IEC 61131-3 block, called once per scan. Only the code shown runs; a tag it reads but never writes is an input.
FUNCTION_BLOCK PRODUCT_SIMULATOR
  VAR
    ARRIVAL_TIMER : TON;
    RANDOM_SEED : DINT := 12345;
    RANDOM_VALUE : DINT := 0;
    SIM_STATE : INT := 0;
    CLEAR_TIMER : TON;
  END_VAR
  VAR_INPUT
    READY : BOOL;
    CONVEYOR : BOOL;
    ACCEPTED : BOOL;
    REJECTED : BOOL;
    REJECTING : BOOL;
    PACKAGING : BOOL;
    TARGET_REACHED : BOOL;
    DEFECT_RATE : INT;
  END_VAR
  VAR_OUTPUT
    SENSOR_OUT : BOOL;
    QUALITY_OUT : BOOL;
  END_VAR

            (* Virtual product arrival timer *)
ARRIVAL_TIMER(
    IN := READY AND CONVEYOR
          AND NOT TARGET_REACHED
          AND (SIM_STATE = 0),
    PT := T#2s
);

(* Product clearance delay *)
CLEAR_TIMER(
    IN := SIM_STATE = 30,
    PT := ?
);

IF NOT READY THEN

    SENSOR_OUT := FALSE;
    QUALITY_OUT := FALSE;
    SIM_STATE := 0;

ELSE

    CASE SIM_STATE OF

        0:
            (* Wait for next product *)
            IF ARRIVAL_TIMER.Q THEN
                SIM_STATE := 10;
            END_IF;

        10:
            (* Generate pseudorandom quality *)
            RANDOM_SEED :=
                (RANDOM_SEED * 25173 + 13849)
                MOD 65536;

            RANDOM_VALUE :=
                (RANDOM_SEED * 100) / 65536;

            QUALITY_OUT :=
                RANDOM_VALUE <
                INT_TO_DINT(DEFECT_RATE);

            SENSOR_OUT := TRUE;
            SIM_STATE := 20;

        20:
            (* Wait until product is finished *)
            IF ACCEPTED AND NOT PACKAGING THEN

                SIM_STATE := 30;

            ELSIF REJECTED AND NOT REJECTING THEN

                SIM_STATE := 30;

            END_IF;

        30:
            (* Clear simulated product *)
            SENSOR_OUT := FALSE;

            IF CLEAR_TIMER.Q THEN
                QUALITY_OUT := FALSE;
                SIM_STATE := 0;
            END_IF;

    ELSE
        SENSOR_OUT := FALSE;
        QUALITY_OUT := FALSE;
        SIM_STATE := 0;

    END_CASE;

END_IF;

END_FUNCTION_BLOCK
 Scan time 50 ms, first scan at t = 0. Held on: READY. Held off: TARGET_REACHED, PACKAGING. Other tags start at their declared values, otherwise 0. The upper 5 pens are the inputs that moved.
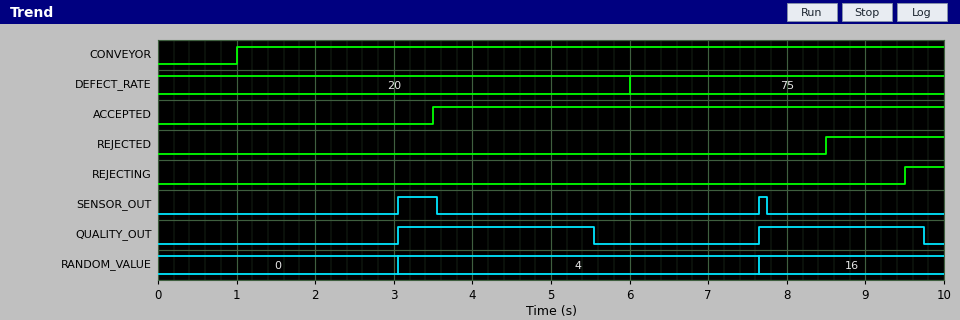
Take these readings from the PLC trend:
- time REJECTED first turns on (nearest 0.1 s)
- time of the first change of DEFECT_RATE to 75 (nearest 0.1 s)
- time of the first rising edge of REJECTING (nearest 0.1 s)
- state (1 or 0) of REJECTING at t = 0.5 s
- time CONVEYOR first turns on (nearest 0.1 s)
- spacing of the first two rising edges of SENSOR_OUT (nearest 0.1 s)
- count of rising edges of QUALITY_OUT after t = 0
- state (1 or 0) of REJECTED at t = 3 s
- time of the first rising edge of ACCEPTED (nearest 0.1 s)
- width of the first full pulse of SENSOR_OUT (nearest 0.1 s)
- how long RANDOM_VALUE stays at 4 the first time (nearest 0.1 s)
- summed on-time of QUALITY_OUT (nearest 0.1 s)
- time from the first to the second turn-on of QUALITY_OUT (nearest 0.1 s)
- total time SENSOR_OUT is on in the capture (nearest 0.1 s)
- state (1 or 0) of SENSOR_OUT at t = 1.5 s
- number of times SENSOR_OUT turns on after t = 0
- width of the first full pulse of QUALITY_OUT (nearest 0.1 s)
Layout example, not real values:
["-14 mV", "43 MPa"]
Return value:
["8.5 s", "6.0 s", "9.5 s", "0", "1.0 s", "4.6 s", "2", "0", "3.5 s", "0.5 s", "4.6 s", "4.6 s", "4.6 s", "0.6 s", "0", "2", "2.5 s"]
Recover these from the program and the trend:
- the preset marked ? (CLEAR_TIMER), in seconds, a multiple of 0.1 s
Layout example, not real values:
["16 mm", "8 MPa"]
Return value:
["2.0 s"]
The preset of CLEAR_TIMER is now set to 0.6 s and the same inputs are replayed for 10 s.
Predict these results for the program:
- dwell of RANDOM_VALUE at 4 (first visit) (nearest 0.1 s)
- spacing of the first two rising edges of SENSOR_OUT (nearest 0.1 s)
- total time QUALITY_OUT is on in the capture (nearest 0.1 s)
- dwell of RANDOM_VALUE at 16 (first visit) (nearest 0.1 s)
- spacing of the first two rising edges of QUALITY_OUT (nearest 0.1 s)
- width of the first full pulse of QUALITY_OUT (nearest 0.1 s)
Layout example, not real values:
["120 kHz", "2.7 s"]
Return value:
["3.2 s", "3.2 s", "2.5 s", "2.8 s", "3.2 s", "1.1 s"]
